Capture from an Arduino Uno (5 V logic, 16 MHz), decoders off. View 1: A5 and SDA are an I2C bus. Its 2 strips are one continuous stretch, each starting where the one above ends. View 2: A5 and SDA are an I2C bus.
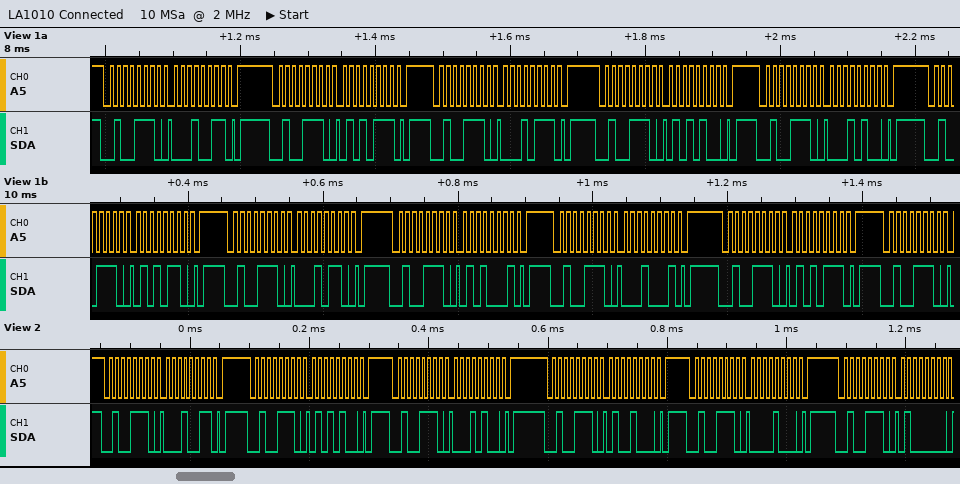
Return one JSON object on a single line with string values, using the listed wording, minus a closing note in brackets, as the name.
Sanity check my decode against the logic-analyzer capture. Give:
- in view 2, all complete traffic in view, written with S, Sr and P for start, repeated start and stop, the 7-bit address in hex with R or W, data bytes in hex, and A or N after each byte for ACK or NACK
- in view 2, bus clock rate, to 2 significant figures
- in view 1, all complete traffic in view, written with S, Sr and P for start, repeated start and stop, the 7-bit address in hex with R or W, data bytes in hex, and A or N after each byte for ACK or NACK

{"in view 2, all complete traffic in view, written with S, Sr and P for start, repeated start and stop, the 7-bit address in hex with R or W, data bytes in hex, and A or N after each byte for ACK or NACK": "S 27W A 13 A P S 27W A 54 A P S 27W A 14 A P S 27W A 48 A P S 27W A 08 A P S 27W A 40 A", "in view 2, bus clock rate, to 2 significant figures": "100 kHz", "in view 1, all complete traffic in view, written with S, Sr and P for start, repeated start and stop, the 7-bit address in hex with R or W, data bytes in hex, and A or N after each byte for ACK or NACK": "S 27W A 13 A P S 27W A 57 A P S 27W A 17 A P S 27W A 54 A P S 27W A 14 A P S 27W A 56 A P S 27W A 16 A P S 27W A 51 A P S 27W A 11 A P S 27W A 57 A P S 27W A"}
